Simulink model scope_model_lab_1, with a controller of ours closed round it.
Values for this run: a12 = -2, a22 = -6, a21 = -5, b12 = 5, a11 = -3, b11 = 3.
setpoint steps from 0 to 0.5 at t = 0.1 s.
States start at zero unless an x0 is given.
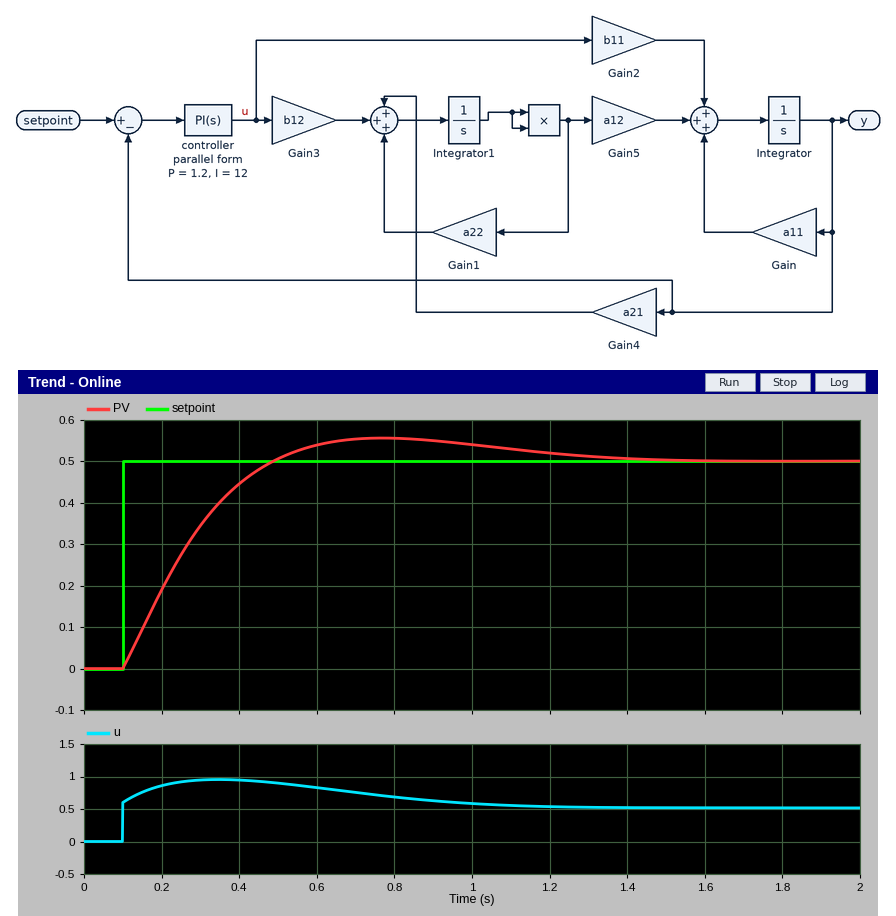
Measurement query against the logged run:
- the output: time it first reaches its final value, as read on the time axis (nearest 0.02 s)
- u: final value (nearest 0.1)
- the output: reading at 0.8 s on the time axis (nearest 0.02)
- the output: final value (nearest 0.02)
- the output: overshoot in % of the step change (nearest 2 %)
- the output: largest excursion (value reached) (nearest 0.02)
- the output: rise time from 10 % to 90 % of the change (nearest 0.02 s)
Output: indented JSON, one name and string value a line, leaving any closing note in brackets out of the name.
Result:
{
  "the output: time it first reaches its final value, as read on the time axis": "0.48 s",
  "u: final value": "0.5",
  "the output: reading at 0.8 s on the time axis": "0.56",
  "the output: final value": "0.50",
  "the output: overshoot in % of the step change": "12 %",
  "the output: largest excursion (value reached)": "0.56",
  "the output: rise time from 10 % to 90 % of the change": "0.28 s"
}
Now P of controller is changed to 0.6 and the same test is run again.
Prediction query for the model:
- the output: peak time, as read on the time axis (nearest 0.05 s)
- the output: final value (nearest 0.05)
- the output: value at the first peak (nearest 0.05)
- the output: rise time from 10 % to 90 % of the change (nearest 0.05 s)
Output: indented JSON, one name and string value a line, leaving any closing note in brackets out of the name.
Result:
{
  "the output: peak time, as read on the time axis": "0.75 s",
  "the output: final value": "0.50",
  "the output: value at the first peak": "0.60",
  "the output: rise time from 10 % to 90 % of the change": "0.25 s"
}
